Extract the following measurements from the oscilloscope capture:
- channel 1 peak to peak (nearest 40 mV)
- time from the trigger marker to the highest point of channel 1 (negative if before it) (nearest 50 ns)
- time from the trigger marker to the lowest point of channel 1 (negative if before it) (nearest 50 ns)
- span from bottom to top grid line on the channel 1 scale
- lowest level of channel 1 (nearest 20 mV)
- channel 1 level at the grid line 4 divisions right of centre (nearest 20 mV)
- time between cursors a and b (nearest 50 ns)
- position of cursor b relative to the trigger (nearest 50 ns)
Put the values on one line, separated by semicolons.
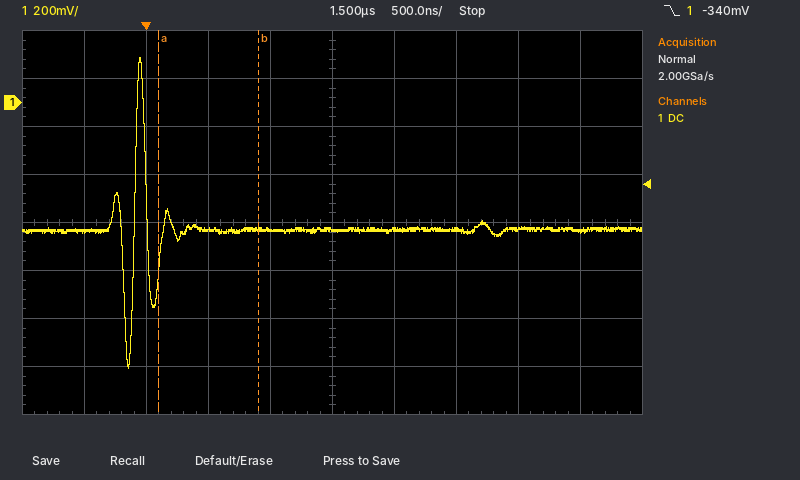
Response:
1.28 V; -50 ns; -150 ns; 1.6 V; -1.10 V; -540 mV; 800 ns; +900 ns
